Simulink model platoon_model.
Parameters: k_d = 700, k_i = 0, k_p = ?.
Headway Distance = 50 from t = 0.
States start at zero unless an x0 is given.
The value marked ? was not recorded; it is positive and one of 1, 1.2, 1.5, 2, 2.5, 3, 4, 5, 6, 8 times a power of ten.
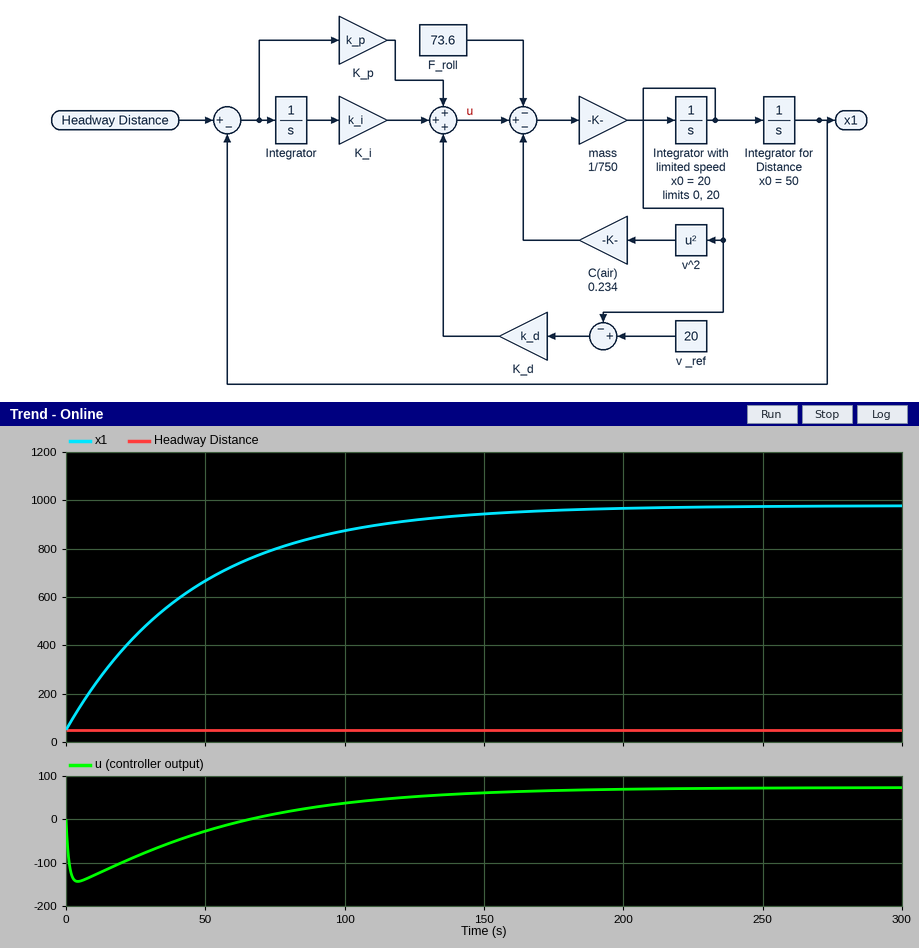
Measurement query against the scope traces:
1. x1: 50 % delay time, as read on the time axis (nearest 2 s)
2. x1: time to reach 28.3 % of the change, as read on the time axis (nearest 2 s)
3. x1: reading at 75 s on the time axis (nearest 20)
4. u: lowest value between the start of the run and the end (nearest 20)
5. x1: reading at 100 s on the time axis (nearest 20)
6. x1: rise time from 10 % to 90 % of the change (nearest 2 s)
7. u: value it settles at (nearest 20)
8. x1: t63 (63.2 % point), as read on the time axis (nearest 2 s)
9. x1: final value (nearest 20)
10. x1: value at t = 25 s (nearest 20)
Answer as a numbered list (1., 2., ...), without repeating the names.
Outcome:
1. 32 s
2. 16 s
3. 800
4. -140
5. 880
6. 100 s
7. 80
8. 46 s
9. 980
10. 440
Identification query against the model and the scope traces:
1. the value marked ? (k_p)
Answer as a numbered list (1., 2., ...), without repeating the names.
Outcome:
1. 15
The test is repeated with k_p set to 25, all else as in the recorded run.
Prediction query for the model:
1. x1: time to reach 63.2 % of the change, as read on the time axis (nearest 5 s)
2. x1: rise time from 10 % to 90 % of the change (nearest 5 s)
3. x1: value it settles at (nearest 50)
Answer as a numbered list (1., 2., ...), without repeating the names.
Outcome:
1. 25 s
2. 60 s
3. 600
